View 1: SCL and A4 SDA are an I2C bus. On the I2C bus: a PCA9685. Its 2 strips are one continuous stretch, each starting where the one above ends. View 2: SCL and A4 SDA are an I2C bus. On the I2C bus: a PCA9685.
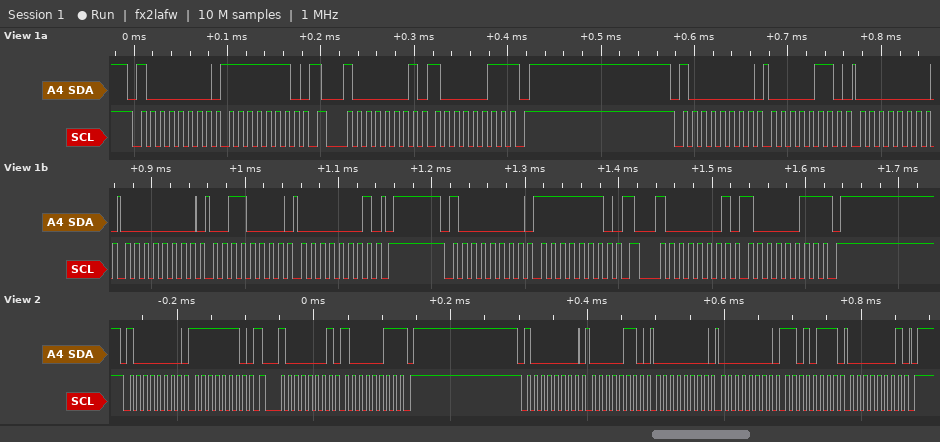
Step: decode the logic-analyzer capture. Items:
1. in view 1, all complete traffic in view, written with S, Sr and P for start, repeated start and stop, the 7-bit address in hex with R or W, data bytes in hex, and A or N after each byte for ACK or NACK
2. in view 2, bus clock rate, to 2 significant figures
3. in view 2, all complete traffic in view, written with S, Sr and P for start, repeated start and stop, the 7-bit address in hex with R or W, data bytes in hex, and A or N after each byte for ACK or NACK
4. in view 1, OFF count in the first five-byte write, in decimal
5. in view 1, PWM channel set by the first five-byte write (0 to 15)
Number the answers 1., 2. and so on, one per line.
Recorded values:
1. S 40W A FE A Sr 40R A 83 N P S 40W A 06 A 00 A 00 A 30 A 01 A P S 40W A FE A Sr 40R A 83 N P
2. 100 kHz
3. S 40W A FE A Sr 40R A 83 N P S 40W A 06 A 00 A 00 A D7 A 01 A P
4. 304
5. 0
